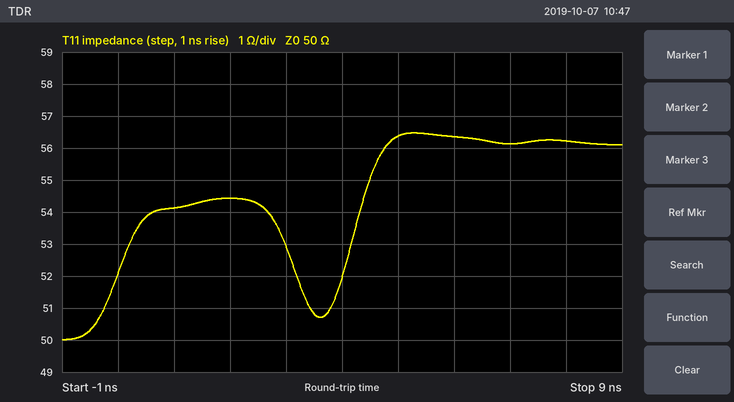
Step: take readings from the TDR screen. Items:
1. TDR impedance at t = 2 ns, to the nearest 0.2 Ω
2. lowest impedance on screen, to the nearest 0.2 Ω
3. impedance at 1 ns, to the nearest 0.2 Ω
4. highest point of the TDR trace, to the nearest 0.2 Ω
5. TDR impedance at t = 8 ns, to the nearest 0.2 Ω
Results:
54.4 Ω
50.0 Ω
54.2 Ω
56.4 Ω
56.2 Ω
